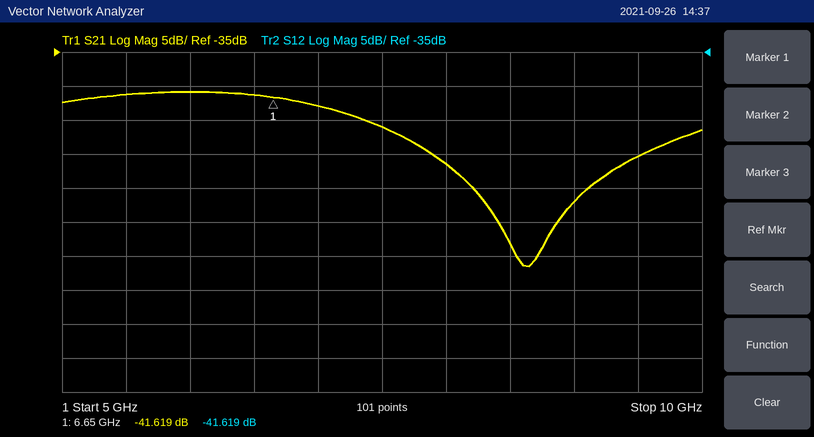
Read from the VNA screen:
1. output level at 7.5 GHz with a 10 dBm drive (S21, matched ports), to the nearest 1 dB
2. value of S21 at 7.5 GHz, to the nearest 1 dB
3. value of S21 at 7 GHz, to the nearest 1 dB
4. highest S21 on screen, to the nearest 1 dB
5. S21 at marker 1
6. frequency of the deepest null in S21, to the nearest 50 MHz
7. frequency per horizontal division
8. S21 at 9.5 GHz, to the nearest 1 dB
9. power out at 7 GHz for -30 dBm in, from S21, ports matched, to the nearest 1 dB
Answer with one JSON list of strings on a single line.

["-36 dBm", "-46 dB", "-43 dB", "-41 dB", "-41.619 dB", "8.65 GHz", "500 MHz", "-50 dB", "-73 dBm"]
